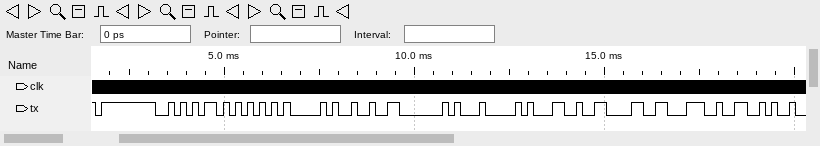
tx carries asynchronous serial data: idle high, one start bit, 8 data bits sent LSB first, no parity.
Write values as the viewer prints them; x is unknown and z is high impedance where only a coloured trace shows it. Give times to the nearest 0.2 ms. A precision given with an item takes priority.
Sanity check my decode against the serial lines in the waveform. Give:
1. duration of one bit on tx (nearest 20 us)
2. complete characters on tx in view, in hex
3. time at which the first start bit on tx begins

160 us
FF, AA, 55, 41, 92, 40, 04, 31, 86, C6, 32
1.6 ms
